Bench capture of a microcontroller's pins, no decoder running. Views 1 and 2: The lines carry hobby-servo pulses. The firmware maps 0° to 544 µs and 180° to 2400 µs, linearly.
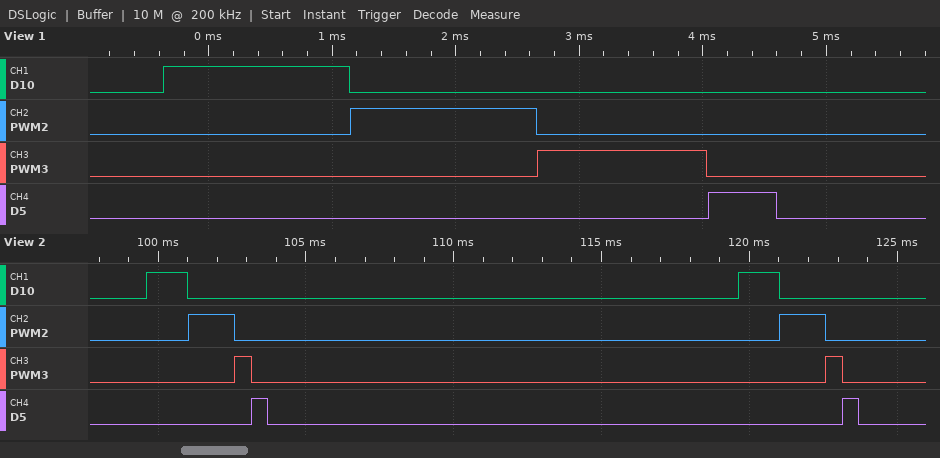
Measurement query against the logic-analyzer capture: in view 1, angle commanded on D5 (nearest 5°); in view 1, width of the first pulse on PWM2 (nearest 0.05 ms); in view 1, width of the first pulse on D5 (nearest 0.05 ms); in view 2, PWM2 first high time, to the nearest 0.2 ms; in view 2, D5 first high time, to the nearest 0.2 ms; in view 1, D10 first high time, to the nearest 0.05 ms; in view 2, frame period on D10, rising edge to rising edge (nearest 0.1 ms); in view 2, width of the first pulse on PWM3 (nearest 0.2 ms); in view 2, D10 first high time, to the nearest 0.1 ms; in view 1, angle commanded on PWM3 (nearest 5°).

0°
1.50 ms
0.55 ms
1.6 ms
0.6 ms
1.50 ms
20.0 ms
0.6 ms
1.4 ms
80°
